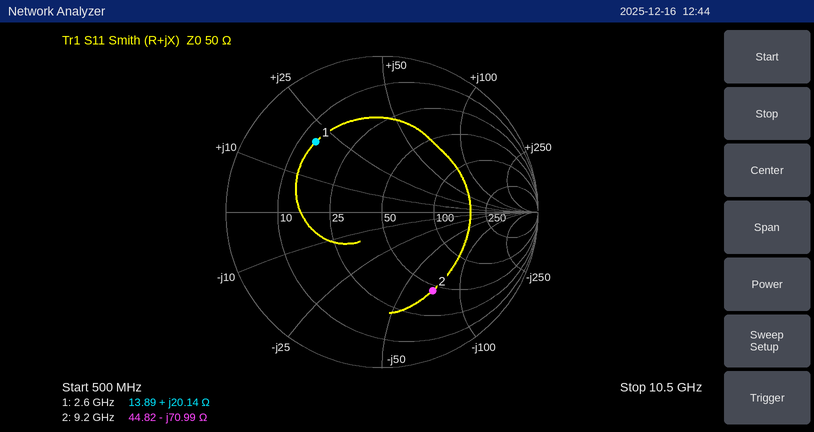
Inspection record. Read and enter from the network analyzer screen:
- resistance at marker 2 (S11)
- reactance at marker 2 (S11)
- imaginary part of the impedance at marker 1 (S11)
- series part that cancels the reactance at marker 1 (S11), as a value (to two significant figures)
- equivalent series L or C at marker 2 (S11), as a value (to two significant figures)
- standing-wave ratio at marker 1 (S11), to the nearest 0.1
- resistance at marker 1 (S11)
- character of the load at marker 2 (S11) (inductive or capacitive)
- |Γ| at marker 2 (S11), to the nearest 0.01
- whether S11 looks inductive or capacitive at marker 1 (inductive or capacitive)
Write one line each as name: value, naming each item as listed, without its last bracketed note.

resistance at marker 2: 44.82 Ω
reactance at marker 2: -70.99 Ω
imaginary part of the impedance at marker 1: +20.14 Ω
series part that cancels the reactance at marker 1 (S11), as a value: 3.0 pF
equivalent series L or C at marker 2 (S11), as a value: 240 fF
standing-wave ratio at marker 1 (S11), to the nearest 0.1: 4.2
resistance at marker 1: 13.89 Ω
character of the load at marker 2 (S11): capacitive
|Γ| at marker 2 (S11), to the nearest 0.01: 0.60
whether S11 looks inductive or capacitive at marker 1: inductive
